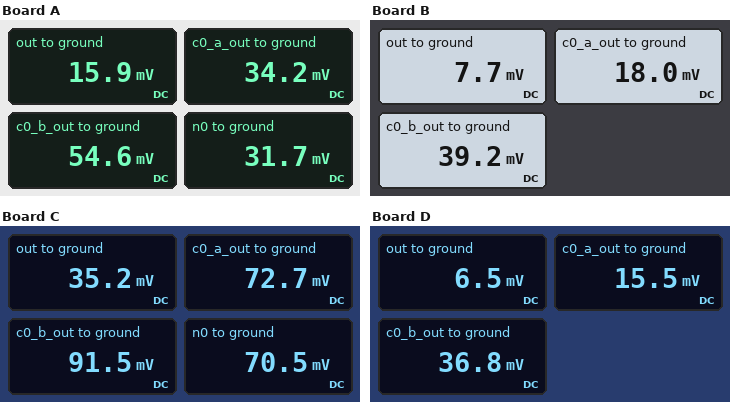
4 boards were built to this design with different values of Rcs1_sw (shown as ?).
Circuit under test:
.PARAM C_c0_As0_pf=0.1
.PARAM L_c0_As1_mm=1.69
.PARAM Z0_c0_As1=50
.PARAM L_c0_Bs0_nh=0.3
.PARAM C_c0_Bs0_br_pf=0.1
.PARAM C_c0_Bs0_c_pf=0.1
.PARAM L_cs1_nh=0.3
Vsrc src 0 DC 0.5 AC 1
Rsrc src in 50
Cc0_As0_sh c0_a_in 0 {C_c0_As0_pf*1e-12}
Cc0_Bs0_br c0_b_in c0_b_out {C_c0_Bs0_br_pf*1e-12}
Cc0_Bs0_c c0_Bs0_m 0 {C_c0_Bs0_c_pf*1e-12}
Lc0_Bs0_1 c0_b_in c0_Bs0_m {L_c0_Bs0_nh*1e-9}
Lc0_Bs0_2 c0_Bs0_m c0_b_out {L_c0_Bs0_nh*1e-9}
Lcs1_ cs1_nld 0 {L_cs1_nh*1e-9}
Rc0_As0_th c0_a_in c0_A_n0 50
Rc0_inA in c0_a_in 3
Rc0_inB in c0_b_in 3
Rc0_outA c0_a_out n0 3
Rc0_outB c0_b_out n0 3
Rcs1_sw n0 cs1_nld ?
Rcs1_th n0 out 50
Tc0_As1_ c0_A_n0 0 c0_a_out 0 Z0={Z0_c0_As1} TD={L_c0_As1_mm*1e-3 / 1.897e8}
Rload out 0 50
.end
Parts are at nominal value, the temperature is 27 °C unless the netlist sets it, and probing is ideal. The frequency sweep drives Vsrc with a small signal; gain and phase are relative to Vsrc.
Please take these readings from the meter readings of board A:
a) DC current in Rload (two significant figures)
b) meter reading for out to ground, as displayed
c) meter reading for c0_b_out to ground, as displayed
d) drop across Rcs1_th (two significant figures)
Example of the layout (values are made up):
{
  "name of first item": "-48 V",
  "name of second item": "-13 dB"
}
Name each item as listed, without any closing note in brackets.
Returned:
{
  "DC current in Rload": "320 µA",
  "meter reading for out to ground, as displayed": "15.9 mV",
  "meter reading for c0_b_out to ground, as displayed": "54.6 mV",
  "drop across Rcs1_th": "16 mV"
}
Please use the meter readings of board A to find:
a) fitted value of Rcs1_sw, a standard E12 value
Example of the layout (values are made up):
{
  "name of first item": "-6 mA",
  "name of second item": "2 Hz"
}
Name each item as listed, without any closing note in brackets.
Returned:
{
  "fitted value of Rcs1_sw, a standard E12 value": "3.9 Ω"
}
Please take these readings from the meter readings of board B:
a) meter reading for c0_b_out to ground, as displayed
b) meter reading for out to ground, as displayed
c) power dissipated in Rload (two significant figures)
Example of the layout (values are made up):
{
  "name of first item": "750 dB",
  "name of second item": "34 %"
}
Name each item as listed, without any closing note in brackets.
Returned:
{
  "meter reading for c0_b_out to ground, as displayed": "39.2 mV",
  "meter reading for out to ground, as displayed": "7.7 mV",
  "power dissipated in Rload": "1.2 µW"
}
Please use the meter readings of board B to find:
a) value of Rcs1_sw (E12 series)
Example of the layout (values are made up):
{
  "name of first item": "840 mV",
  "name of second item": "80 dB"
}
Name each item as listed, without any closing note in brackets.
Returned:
{
  "value of Rcs1_sw": "1.8 Ω"
}
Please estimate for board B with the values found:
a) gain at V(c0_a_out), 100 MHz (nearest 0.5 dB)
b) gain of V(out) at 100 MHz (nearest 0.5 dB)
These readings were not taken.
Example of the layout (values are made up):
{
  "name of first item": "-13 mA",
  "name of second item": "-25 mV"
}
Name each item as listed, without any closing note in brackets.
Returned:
{
  "gain at V(c0_a_out), 100 MHz": "-29.0 dB",
  "gain of V(out) at 100 MHz": "-36.0 dB"
}
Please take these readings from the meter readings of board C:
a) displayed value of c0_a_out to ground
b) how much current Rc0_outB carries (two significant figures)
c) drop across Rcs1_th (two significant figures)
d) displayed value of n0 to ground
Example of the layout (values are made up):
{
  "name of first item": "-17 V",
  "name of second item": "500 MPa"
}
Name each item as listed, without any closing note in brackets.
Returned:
{
  "displayed value of c0_a_out to ground": "72.7 mV",
  "how much current Rc0_outB carries": "7.0 mA",
  "drop across Rcs1_th": "35 mV",
  "displayed value of n0 to ground": "70.5 mV"
}
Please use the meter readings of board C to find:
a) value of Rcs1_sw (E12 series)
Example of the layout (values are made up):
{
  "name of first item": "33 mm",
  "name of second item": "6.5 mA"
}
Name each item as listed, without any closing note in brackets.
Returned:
{
  "value of Rcs1_sw": "10 Ω"
}
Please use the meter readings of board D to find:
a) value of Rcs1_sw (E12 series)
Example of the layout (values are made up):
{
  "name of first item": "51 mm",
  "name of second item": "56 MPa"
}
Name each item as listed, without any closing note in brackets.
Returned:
{
  "value of Rcs1_sw": "1.5 Ω"
}
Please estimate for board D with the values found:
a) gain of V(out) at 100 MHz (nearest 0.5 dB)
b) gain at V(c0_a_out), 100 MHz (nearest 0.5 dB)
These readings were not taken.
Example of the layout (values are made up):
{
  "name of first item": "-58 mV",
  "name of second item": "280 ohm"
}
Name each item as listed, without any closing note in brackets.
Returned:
{
  "gain of V(out) at 100 MHz": "-37.5 dB",
  "gain at V(c0_a_out), 100 MHz": "-30.0 dB"
}
